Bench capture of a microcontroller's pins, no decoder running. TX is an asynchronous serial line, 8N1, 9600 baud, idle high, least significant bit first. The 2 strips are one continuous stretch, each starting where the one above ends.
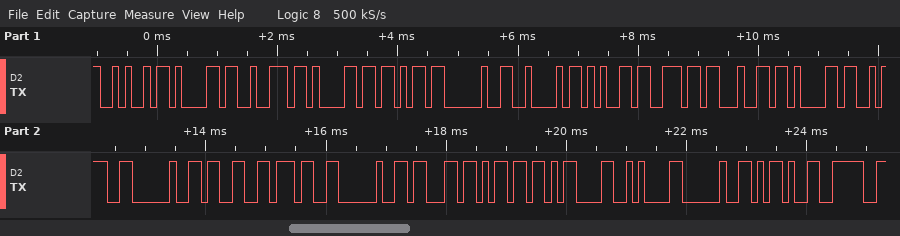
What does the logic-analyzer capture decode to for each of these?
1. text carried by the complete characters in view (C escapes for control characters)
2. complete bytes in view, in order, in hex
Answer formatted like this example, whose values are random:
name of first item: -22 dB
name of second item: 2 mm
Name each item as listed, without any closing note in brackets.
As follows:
text carried by the complete characters in view: "Jarak Benda: 37 cm\r\n ->"
complete bytes in view, in order, in hex: 4A 61 72 61 6B 20 42 65 6E 64 61 3A 20 33 37 20 63 6D 0D 0A 20 2D 3E
